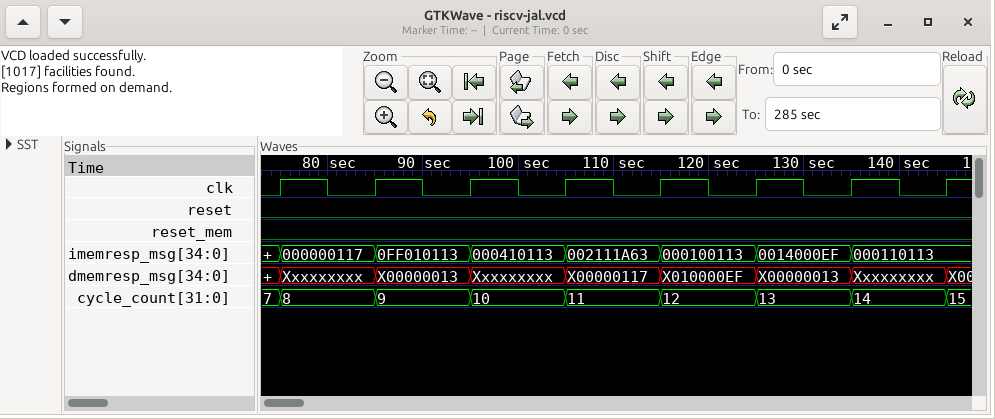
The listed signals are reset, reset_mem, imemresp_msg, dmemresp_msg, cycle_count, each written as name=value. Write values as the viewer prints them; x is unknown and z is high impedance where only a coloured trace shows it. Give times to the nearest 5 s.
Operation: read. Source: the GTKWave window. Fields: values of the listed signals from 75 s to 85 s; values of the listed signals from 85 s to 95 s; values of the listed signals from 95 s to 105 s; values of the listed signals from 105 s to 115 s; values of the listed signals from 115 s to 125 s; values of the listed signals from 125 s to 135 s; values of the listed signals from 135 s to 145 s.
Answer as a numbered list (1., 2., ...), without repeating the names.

1. reset=0, reset_mem=0, imemresp_msg=000000117, dmemresp_msg=Xxxxxxxxx, cycle_count=8
2. reset=0, reset_mem=0, imemresp_msg=0FF010113, dmemresp_msg=X00000013, cycle_count=9
3. reset=0, reset_mem=0, imemresp_msg=000410113, dmemresp_msg=Xxxxxxxxx, cycle_count=10
4. reset=0, reset_mem=0, imemresp_msg=002111A63, dmemresp_msg=X00000117, cycle_count=11
5. reset=0, reset_mem=0, imemresp_msg=000100113, dmemresp_msg=X010000EF, cycle_count=12
6. reset=0, reset_mem=0, imemresp_msg=0014000EF, dmemresp_msg=X00000013, cycle_count=13
7. reset=0, reset_mem=0, imemresp_msg=000110113, dmemresp_msg=Xxxxxxxxx, cycle_count=14
